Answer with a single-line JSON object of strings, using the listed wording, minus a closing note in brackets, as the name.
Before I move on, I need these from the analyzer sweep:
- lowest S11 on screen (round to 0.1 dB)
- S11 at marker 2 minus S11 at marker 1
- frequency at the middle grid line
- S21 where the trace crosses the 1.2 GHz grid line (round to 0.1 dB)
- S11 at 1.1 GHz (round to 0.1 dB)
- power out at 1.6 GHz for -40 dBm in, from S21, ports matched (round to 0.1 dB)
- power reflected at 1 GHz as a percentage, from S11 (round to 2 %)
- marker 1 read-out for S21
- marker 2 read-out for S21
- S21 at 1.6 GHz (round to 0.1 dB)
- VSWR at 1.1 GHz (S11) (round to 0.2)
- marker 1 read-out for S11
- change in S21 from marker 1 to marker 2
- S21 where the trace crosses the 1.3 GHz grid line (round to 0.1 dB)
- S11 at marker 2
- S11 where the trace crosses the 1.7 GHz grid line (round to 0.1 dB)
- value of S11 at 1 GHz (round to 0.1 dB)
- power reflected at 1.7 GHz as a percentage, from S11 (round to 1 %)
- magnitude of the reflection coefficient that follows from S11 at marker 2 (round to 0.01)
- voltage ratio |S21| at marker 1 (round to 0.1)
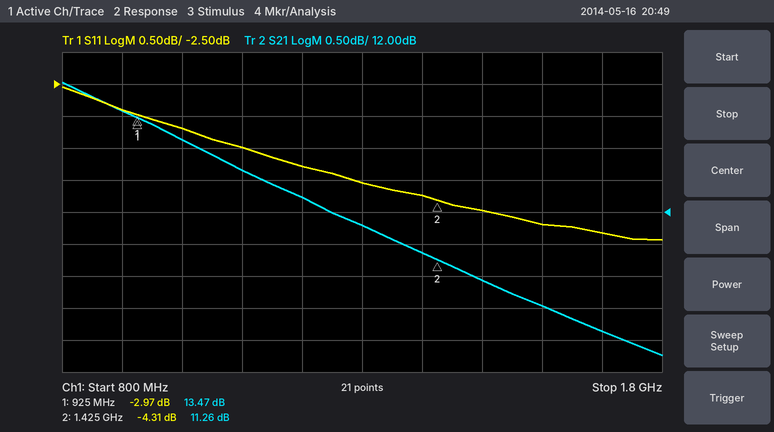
{"lowest S11 on screen": "-4.9 dB", "S11 at marker 2 minus S11 at marker 1": "-1.34 dB", "frequency at the middle grid line": "1.3 GHz", "S21 where the trace crosses the 1.2 GHz grid line": "12.2 dB", "S11 at 1.1 GHz": "-3.5 dB", "power out at 1.6 GHz for -40 dBm in, from S21, ports matched": "-29.5 dBm", "power reflected at 1 GHz as a percentage, from S11": "48 %", "marker 1 read-out for S21": "13.47 dB", "marker 2 read-out for S21": "11.26 dB", "S21 at 1.6 GHz": "10.5 dB", "VSWR at 1.1 GHz (S11)": "5.0", "marker 1 read-out for S11": "-2.97 dB", "change in S21 from marker 1 to marker 2": "-2.21 dB", "S21 where the trace crosses the 1.3 GHz grid line": "11.8 dB", "S11 at marker 2": "-4.31 dB", "S11 where the trace crosses the 1.7 GHz grid line": "-4.8 dB", "value of S11 at 1 GHz": "-3.2 dB", "power reflected at 1.7 GHz as a percentage, from S11": "33 %", "magnitude of the reflection coefficient that follows from S11 at marker 2": "0.61", "voltage ratio |S21| at marker 1": "4.7"}
